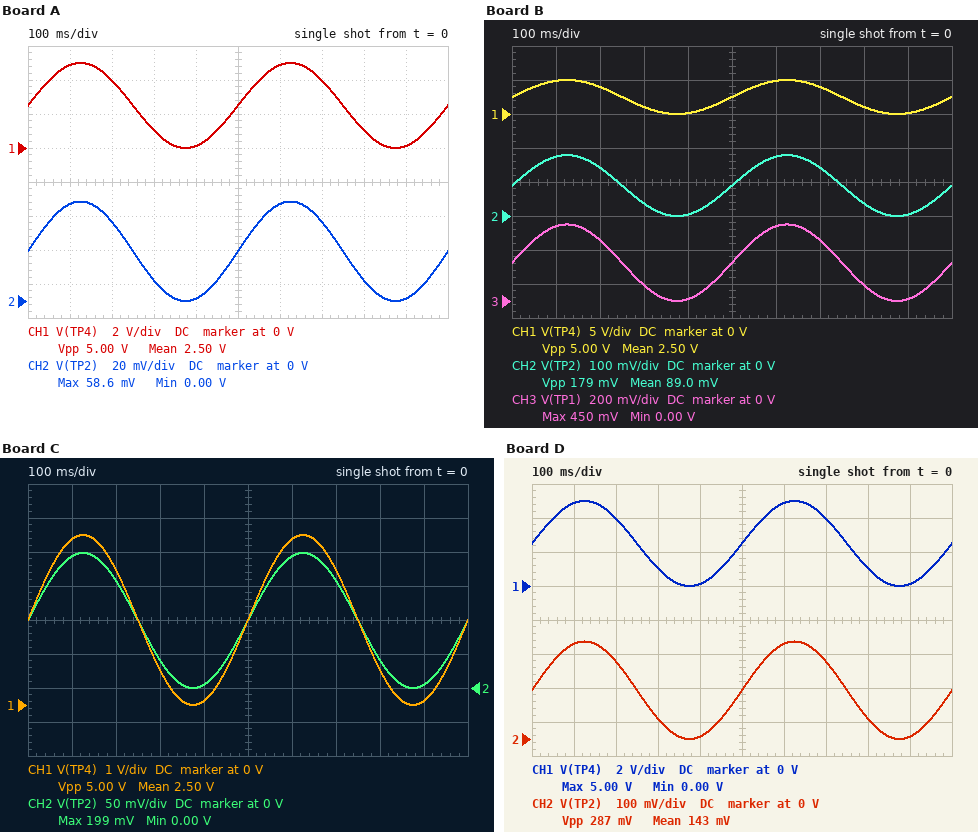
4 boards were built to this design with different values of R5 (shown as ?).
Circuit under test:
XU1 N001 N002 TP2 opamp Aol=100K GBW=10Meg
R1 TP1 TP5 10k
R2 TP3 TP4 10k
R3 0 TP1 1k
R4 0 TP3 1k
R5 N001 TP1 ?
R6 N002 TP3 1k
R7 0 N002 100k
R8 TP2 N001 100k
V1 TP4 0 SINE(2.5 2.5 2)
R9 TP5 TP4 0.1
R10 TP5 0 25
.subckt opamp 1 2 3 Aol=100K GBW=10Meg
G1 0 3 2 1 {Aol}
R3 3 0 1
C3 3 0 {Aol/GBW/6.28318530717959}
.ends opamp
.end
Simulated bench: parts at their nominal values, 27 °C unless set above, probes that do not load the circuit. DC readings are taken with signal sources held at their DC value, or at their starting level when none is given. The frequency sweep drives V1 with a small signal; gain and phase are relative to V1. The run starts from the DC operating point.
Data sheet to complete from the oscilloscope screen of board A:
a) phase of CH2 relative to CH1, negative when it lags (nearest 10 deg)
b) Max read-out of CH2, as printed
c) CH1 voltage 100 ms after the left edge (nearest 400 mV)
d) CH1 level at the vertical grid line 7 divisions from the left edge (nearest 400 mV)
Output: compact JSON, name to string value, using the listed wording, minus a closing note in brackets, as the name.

{"phase of CH2 relative to CH1, negative when it lags": "0 deg", "Max read-out of CH2, as printed": "58.6 mV", "CH1 voltage 100 ms after the left edge": "4.8 V", "CH1 level at the vertical grid line 7 divisions from the left edge": "4.0 V"}
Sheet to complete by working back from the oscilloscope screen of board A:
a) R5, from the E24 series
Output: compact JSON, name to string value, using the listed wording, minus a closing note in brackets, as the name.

{"R5, from the E24 series": "820 Ω"}
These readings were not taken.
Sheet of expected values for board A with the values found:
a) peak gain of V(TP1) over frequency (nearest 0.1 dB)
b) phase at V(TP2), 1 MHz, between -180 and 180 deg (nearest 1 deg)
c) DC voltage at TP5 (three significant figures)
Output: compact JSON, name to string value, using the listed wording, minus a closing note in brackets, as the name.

{"peak gain of V(TP1) over frequency": "-20.9 dB", "phase at V(TP2), 1 MHz, between -180 and 180 deg": "-80 deg", "DC voltage at TP5": "2.49 V"}
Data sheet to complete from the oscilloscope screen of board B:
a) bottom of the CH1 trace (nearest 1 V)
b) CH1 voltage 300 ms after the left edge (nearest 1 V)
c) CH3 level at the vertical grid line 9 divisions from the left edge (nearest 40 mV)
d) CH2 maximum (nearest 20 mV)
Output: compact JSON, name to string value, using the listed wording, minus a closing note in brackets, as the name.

{"bottom of the CH1 trace": "0 V", "CH1 voltage 300 ms after the left edge": "1 V", "CH3 level at the vertical grid line 9 divisions from the left edge": "0 V", "CH2 maximum": "180 mV"}
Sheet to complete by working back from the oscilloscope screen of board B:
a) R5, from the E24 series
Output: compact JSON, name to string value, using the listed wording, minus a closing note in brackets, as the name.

{"R5, from the E24 series": "1.6 kΩ"}
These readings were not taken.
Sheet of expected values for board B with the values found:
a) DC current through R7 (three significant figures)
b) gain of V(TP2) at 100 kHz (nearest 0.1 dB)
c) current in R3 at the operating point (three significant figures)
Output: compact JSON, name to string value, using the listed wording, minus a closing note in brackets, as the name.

{"DC current through R7": "2.23 µA", "gain of V(TP2) at 100 kHz": "-29.6 dB", "current in R3 at the operating point": "225 µA"}
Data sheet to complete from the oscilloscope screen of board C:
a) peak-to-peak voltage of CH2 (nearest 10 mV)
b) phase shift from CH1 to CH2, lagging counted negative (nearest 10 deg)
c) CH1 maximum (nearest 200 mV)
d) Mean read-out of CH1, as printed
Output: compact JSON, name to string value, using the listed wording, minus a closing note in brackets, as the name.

{"peak-to-peak voltage of CH2": "200 mV", "phase shift from CH1 to CH2, lagging counted negative": "0 deg", "CH1 maximum": "5.0 V", "Mean read-out of CH1, as printed": "2.50 V"}
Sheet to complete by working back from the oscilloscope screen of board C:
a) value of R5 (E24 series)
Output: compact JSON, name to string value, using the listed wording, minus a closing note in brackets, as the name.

{"value of R5": "1.8 kΩ"}
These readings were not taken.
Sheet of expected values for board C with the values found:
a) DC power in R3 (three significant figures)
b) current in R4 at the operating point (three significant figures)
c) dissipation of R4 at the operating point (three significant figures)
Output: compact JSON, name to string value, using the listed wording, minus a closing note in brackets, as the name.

{"DC power in R3": "50.7 µW", "current in R4 at the operating point": "225 µA", "dissipation of R4 at the operating point": "50.7 µW"}
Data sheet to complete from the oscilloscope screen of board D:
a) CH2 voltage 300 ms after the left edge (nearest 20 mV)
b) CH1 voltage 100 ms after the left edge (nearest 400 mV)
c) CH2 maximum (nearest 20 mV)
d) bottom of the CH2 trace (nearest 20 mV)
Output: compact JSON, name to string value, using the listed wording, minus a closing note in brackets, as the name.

{"CH2 voltage 300 ms after the left edge": "60 mV", "CH1 voltage 100 ms after the left edge": "4.8 V", "CH2 maximum": "280 mV", "bottom of the CH2 trace": "0 V"}
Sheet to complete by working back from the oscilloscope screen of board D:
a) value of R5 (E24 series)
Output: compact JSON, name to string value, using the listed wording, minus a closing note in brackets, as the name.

{"value of R5": "3.3 kΩ"}
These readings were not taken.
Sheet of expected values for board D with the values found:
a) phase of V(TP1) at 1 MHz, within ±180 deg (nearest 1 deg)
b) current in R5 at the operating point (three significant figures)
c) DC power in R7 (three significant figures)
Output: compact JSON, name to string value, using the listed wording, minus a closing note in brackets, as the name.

{"phase of V(TP1) at 1 MHz, within ±180 deg": "0 deg", "current in R5 at the operating point": "796 nA", "DC power in R7": "497 nW"}
